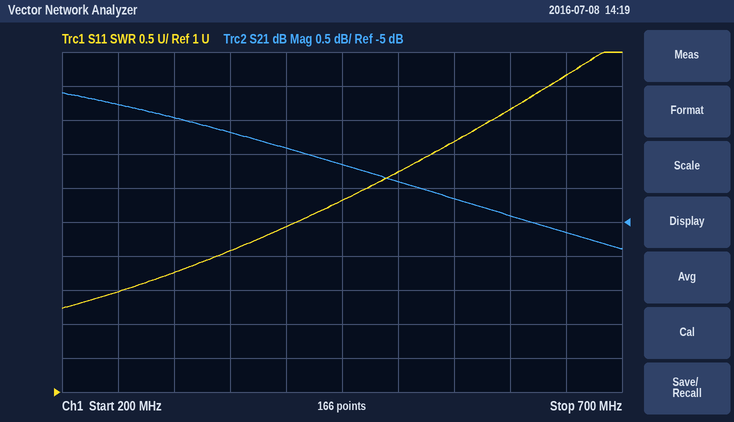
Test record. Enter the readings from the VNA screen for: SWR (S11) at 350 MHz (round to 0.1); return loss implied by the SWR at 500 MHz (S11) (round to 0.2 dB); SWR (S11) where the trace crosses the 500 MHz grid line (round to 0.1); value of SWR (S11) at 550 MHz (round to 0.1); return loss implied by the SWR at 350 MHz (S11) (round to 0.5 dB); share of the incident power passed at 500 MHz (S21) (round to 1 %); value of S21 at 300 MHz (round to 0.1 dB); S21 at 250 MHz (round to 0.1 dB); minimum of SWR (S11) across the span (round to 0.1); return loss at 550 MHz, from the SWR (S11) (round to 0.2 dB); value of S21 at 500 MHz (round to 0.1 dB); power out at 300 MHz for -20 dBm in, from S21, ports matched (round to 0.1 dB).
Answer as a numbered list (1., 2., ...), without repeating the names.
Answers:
1. 3.1
2. 4.2 dB
3. 4.2
4. 4.7
5. 6.0 dB
6. 36 %
7. -3.5 dB
8. -3.3 dB
9. 2.2
10. 3.8 dB
11. -4.4 dB
12. -23.5 dBm
